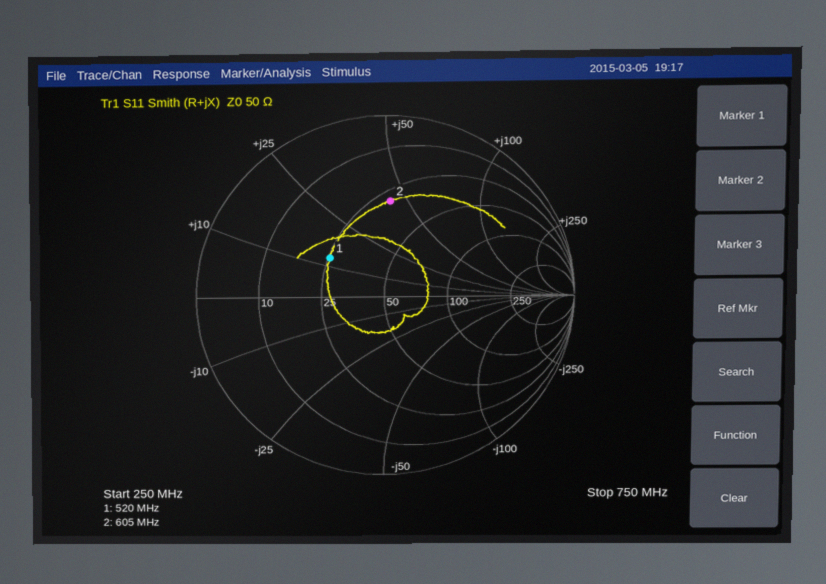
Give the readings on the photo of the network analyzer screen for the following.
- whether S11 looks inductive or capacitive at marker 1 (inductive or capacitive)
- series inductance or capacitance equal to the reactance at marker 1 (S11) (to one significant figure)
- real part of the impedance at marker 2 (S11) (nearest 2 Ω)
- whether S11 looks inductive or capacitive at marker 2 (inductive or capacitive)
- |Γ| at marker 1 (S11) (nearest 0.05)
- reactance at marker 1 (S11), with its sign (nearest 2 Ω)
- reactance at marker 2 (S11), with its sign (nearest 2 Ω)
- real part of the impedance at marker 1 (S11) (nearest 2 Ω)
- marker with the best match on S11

inductive
4 nH
30 Ω
inductive
0.35
+12 Ω
+44 Ω
26 Ω
marker 1
